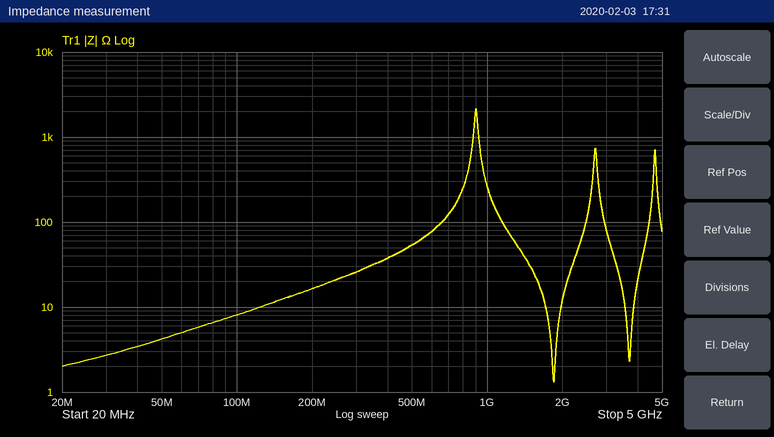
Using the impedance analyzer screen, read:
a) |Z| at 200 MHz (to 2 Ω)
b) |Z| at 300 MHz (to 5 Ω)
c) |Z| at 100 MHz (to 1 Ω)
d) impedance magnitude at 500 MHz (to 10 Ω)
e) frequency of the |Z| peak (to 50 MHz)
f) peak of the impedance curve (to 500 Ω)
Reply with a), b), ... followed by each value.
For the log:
a) 16 Ω
b) 25 Ω
c) 8 Ω
d) 50 Ω
e) 900 MHz
f) 2.0 kΩ
